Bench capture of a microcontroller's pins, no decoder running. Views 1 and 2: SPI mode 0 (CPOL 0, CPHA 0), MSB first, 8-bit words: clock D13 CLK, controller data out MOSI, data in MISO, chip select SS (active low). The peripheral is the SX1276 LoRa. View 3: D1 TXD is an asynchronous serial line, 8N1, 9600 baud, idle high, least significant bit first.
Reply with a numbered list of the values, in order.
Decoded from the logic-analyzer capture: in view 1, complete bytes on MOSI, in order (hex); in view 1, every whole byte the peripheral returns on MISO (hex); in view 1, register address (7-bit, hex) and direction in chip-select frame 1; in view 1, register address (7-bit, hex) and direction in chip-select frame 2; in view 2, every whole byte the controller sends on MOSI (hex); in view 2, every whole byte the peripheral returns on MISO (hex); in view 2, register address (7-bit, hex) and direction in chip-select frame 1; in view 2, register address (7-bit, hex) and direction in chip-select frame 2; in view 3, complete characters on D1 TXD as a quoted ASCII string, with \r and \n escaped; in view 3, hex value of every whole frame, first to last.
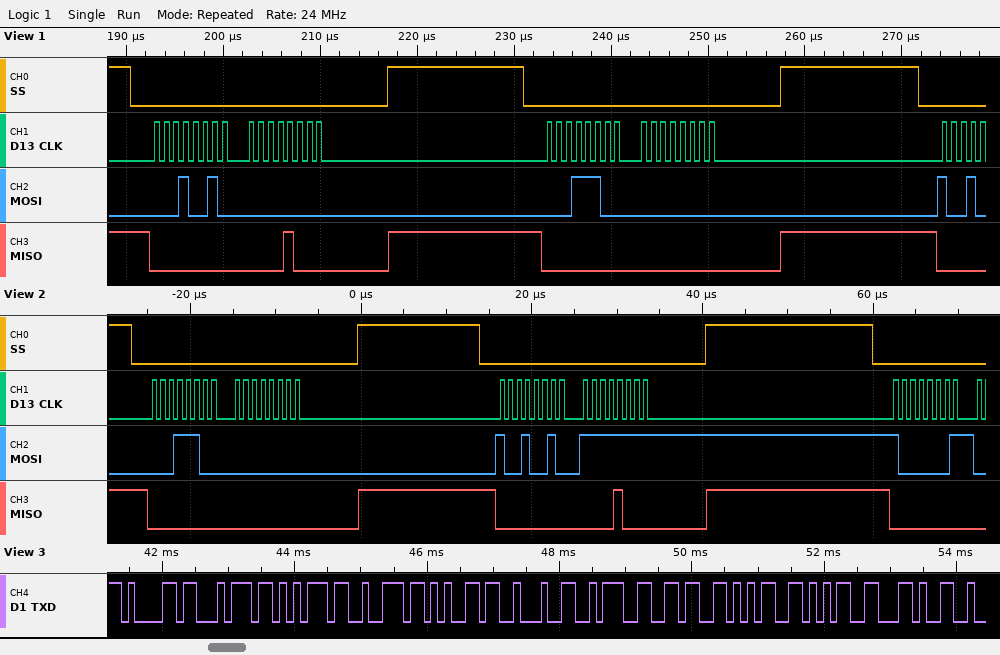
1. 0x12 0x00 0x1C 0x00
2. 0x00 0x08 0x00 0x00
3. 0x12 read
4. 0x1C read
5. 0x1C 0x00 0x92 0xFF 0x81
6. 0x00 0x00 0x00 0x08 0x00
7. 0x1C read
8. 0x12 write
9. "ature\":655,"
10. 61 74 75 72 65 22 3A 36 35 35 2C
